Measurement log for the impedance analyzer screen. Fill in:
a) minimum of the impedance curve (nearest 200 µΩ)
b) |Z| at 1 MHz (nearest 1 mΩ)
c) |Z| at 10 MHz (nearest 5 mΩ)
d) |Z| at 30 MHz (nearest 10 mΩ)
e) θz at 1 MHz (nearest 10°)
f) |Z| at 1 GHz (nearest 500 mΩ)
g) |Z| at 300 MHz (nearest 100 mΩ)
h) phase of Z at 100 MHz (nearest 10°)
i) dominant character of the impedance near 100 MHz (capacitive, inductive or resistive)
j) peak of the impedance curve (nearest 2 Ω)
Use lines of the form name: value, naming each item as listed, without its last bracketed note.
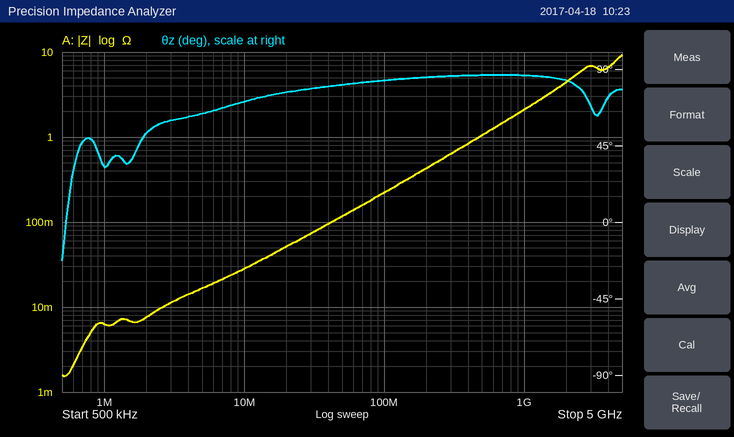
minimum of the impedance curve: 1.6 mΩ
|Z| at 1 MHz: 6 mΩ
|Z| at 10 MHz: 30 mΩ
|Z| at 30 MHz: 70 mΩ
θz at 1 MHz: 30°
|Z| at 1 GHz: 2.0 Ω
|Z| at 300 MHz: 600 mΩ
phase of Z at 100 MHz: 80°
dominant character of the impedance near 100 MHz: inductive
peak of the impedance curve: 10 Ω
